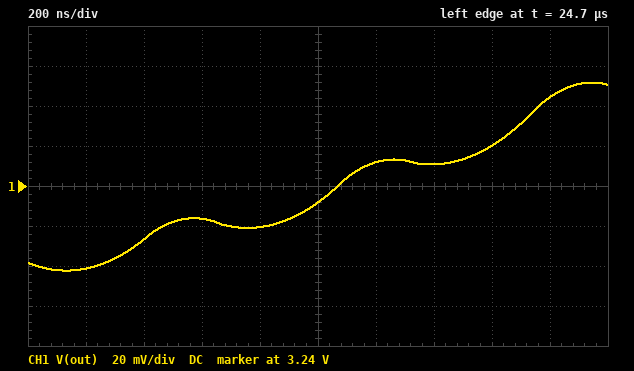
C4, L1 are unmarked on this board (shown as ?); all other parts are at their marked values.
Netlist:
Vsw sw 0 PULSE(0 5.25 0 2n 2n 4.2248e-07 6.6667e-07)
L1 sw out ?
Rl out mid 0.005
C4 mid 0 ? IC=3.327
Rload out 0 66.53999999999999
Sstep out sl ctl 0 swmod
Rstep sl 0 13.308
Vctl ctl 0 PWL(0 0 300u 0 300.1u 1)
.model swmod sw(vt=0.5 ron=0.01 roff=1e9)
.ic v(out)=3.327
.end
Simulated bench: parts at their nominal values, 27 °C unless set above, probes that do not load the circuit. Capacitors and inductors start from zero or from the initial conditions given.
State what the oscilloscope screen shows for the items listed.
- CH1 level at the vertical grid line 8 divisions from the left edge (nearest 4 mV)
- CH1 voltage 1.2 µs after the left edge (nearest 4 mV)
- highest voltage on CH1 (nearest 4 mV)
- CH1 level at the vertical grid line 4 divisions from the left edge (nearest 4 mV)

3.260 V
3.252 V
3.292 V
3.220 V
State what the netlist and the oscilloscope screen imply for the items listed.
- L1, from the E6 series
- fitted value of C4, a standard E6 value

1 µH
4.7 µF
